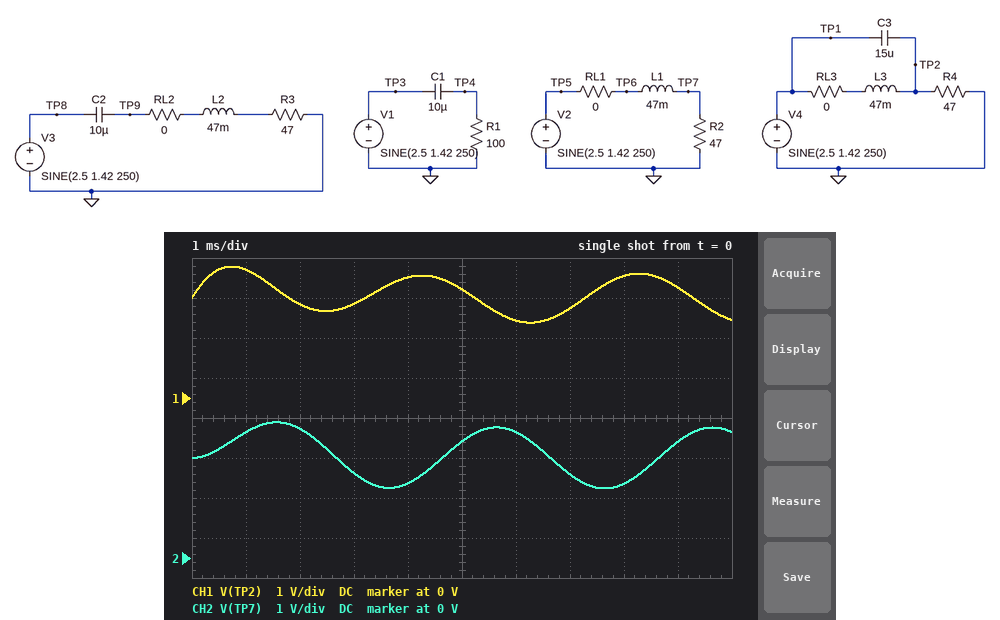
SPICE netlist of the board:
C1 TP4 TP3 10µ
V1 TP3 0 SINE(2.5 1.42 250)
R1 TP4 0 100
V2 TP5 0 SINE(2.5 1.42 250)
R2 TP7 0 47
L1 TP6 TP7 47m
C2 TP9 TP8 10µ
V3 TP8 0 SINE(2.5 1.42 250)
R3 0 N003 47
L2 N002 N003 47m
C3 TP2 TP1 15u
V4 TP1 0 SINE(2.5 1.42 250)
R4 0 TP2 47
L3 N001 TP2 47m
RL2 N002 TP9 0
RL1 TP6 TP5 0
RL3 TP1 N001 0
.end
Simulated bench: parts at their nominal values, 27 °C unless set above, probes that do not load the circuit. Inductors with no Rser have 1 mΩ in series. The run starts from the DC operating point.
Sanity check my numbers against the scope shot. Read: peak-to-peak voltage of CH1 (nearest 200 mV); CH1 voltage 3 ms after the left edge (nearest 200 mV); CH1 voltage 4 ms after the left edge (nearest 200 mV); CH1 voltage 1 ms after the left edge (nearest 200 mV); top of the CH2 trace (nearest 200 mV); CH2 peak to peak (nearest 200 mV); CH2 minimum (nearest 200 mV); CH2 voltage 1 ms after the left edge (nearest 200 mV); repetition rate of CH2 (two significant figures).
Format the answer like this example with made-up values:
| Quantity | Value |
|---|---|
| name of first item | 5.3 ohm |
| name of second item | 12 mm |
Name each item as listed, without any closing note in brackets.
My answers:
| Quantity | Value |
|---|---|
| peak-to-peak voltage of CH1 | 1.4 V |
| CH1 voltage 3 ms after the left edge | 2.4 V |
| CH1 voltage 4 ms after the left edge | 3.0 V |
| CH1 voltage 1 ms after the left edge | 3.2 V |
| top of the CH2 trace | 3.4 V |
| CH2 peak to peak | 1.6 V |
| CH2 minimum | 1.8 V |
| CH2 voltage 1 ms after the left edge | 3.2 V |
| repetition rate of CH2 | 250 Hz |
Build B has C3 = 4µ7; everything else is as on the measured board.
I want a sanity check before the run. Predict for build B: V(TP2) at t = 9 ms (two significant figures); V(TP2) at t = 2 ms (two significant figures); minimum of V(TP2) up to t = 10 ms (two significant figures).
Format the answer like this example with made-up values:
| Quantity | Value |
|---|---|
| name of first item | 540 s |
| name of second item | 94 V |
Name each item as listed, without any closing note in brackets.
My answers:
| Quantity | Value |
|---|---|
| V(TP2) at t = 9 ms | 2.6 V |
| V(TP2) at t = 2 ms | 3.0 V |
| minimum of V(TP2) up to t = 10 ms | 2.1 V |
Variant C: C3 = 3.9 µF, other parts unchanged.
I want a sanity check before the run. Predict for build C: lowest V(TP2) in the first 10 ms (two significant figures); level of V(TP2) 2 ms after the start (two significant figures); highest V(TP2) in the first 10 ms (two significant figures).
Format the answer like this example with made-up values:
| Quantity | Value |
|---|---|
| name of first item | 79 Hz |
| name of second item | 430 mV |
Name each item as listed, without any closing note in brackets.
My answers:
| Quantity | Value |
|---|---|
| lowest V(TP2) in the first 10 ms | 2.0 V |
| level of V(TP2) 2 ms after the start | 3.0 V |
| highest V(TP2) in the first 10 ms | 3.1 V |
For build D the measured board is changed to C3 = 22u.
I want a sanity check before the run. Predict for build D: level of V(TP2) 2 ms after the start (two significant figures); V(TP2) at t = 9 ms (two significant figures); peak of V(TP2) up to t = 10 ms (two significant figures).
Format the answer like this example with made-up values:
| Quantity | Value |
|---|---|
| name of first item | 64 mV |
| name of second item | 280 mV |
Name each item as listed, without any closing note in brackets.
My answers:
| Quantity | Value |
|---|---|
| level of V(TP2) 2 ms after the start | 2.2 V |
| V(TP2) at t = 9 ms | 3.2 V |
| peak of V(TP2) up to t = 10 ms | 3.5 V |
